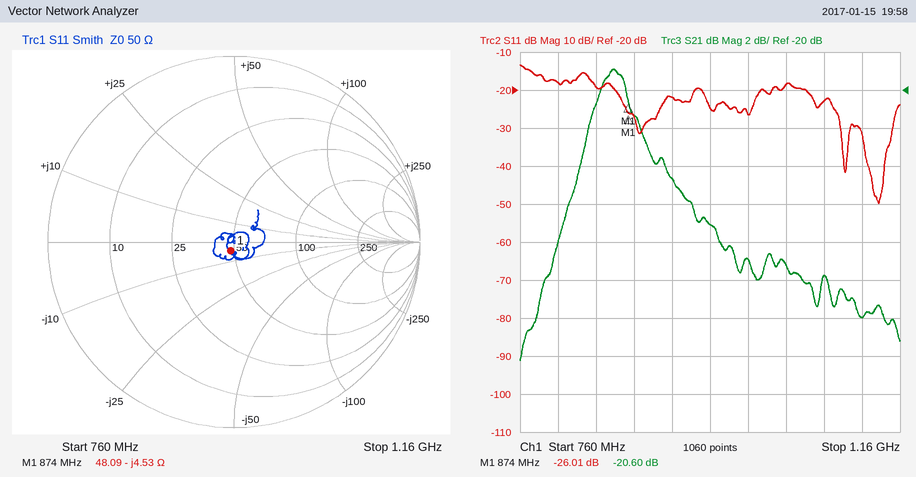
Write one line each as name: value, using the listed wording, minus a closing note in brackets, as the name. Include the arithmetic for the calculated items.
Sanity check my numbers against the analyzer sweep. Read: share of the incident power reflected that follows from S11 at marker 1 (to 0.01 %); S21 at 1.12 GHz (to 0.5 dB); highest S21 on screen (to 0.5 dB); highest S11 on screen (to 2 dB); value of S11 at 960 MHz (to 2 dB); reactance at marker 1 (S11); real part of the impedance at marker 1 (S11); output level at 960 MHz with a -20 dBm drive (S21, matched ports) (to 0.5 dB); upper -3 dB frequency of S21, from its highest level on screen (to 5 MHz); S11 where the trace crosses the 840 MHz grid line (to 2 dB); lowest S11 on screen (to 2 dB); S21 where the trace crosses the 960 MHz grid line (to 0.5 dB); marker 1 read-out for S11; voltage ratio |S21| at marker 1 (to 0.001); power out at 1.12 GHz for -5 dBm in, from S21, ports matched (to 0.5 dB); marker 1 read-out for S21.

share of the incident power reflected that follows from S11 at marker 1: 10^(-26.01/10) ≈ 0.25 %
S21 at 1.12 GHz: -32.0 dB
highest S21 on screen: -19.0 dB
highest S11 on screen: -14 dB
value of S11 at 960 MHz: -24 dB
reactance at marker 1: -4.53 Ω
real part of the impedance at marker 1: 48.09 Ω
output level at 960 MHz with a -20 dBm drive (S21, matched ports): -20 dBm + (-27.0 dB) = -47.0 dBm
upper -3 dB frequency of S21, from its highest level on screen: 885 MHz
S11 where the trace crosses the 840 MHz grid line: -20 dB
lowest S11 on screen: -50 dB
S21 where the trace crosses the 960 MHz grid line: -27.0 dB
marker 1 read-out for S11: -26.01 dB
voltage ratio |S21| at marker 1: 10^(-20.6/20) ≈ 0.093
power out at 1.12 GHz for -5 dBm in, from S21, ports matched: -5 dBm + (-32.0 dB) = -37.0 dBm
marker 1 read-out for S21: -20.60 dB
